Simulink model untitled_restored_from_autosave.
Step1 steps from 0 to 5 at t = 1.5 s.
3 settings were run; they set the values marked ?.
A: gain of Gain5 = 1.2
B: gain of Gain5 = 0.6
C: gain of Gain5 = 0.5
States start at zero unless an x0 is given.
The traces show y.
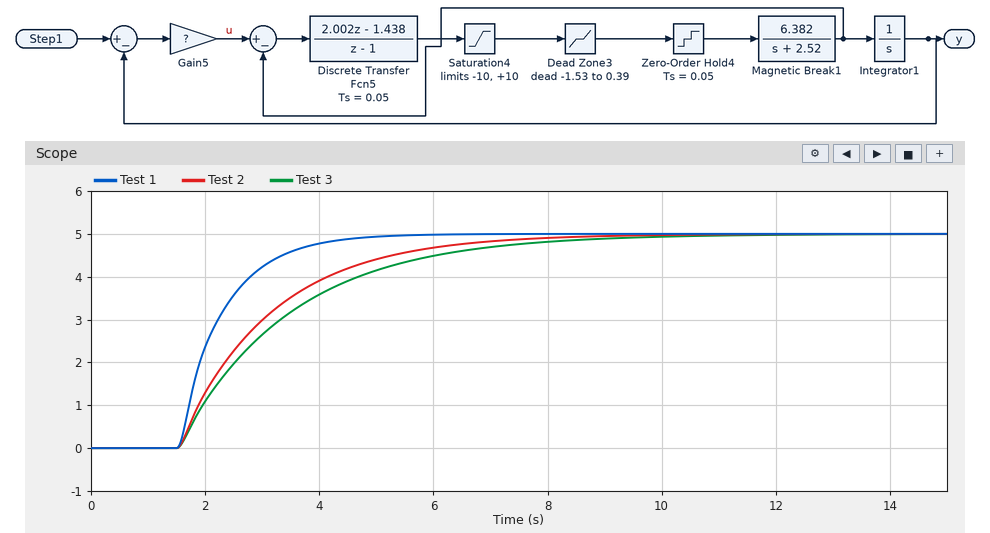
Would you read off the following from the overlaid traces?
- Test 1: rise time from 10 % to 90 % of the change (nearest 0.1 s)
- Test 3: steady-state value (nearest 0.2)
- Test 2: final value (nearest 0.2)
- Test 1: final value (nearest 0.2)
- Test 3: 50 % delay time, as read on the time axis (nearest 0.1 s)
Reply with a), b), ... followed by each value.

a) 1.7 s
b) 5.0
c) 5.0
d) 5.0
e) 2.9 s
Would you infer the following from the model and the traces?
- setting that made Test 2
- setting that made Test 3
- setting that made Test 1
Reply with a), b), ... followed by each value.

a) B
b) C
c) A
